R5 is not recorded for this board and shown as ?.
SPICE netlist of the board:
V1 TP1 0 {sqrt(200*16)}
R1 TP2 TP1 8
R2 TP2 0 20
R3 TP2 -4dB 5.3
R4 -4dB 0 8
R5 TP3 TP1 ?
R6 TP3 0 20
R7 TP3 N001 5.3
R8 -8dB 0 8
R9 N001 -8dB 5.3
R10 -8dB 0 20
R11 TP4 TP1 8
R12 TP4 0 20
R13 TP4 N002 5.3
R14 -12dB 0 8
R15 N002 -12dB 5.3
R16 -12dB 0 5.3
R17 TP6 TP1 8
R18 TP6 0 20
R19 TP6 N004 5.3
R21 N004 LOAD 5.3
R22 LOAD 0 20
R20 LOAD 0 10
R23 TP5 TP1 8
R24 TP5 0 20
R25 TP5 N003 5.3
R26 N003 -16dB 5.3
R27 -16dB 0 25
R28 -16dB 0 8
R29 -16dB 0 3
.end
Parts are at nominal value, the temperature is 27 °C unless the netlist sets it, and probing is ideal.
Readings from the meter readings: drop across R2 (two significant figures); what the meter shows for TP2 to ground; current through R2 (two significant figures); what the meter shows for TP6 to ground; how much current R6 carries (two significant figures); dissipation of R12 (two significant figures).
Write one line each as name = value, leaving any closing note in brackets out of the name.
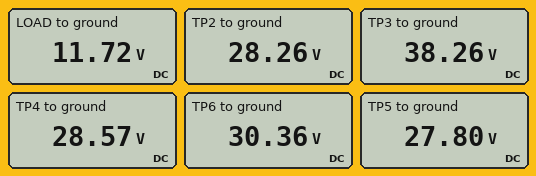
drop across R2 = 28 V
what the meter shows for TP2 to ground = 28.26 V
current through R2 = 1.4 A
what the meter shows for TP6 to ground = 30.36 V
how much current R6 carries = 1.9 A
dissipation of R12 = 41 W
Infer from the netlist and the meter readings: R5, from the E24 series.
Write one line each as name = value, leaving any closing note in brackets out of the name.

R5, from the E24 series = 4.3 Ω
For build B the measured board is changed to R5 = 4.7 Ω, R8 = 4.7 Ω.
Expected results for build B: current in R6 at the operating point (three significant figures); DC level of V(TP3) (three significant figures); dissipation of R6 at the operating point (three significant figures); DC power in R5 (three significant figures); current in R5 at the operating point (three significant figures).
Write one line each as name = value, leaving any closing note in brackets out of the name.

current in R6 at the operating point = 1.81 A
DC level of V(TP3) = 36.2 V
dissipation of R6 at the operating point = 65.6 W
DC power in R5 = 88.0 W
current in R5 at the operating point = 4.33 A
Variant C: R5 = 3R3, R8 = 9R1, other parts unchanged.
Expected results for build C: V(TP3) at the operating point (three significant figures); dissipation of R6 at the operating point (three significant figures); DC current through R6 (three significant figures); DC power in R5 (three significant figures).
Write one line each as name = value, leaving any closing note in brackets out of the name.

V(TP3) at the operating point = 41.6 V
dissipation of R6 at the operating point = 86.4 W
DC current through R6 = 2.08 A
DC power in R5 = 68.2 W
